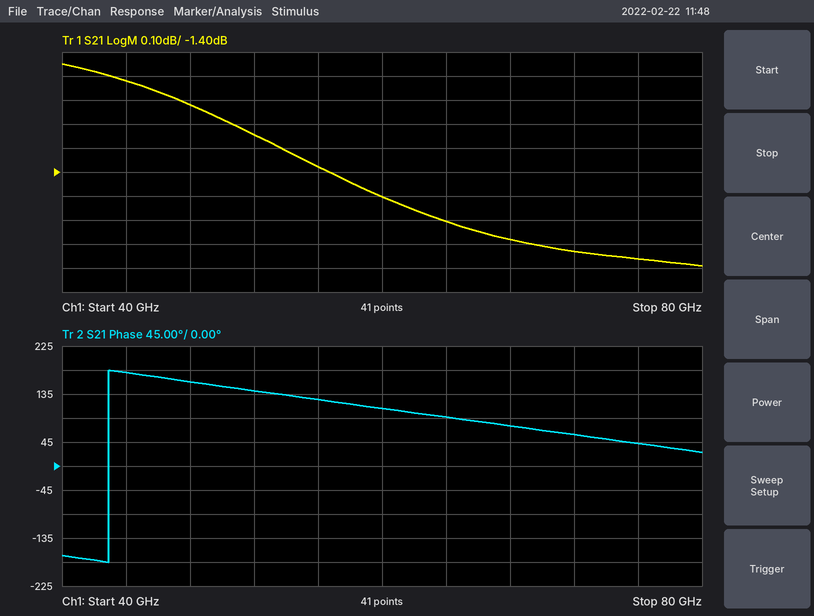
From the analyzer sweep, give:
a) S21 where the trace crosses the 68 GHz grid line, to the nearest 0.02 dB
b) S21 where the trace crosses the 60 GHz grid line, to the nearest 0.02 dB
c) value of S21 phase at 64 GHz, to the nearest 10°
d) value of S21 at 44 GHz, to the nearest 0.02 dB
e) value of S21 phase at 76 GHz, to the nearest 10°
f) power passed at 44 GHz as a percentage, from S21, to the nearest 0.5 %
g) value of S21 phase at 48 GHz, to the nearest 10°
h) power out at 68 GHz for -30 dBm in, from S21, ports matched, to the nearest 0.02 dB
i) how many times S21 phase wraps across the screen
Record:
-1.68 dB
-1.50 dB
90°
-1.02 dB
40°
79.0 %
160°
-31.68 dBm
1
